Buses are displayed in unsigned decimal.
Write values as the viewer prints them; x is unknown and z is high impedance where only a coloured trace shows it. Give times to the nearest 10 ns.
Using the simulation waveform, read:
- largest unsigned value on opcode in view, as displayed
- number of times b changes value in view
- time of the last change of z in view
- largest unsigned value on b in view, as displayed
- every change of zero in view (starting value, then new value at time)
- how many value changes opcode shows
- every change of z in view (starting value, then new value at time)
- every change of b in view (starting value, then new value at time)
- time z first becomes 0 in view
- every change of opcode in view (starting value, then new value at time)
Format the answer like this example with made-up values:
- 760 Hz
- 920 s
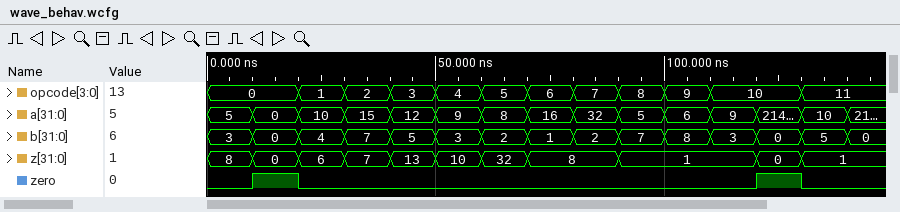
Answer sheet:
- 11
- 14
- 130 ns
- 8
- 0, 1 at 10 ns, 0 at 20 ns, 1 at 120 ns, 0 at 130 ns
- 11
- 8, 0 at 10 ns, 6 at 20 ns, 7 at 30 ns, 13 at 40 ns, 10 at 50 ns, 32 at 60 ns, 8 at 70 ns, 1 at 90 ns, 0 at 120 ns, 1 at 130 ns
- 3, 0 at 10 ns, 4 at 20 ns, 7 at 30 ns, 5 at 40 ns, 3 at 50 ns, 2 at 60 ns, 1 at 70 ns, 2 at 80 ns, 7 at 90 ns, 8 at 100 ns, 3 at 110 ns, 0 at 120 ns, 5 at 130 ns, 0 at 140 ns
- 10 ns
- 0, 1 at 20 ns, 2 at 30 ns, 3 at 40 ns, 4 at 50 ns, 5 at 60 ns, 6 at 70 ns, 7 at 80 ns, 8 at 90 ns, 9 at 100 ns, 10 at 110 ns, 11 at 130 ns
